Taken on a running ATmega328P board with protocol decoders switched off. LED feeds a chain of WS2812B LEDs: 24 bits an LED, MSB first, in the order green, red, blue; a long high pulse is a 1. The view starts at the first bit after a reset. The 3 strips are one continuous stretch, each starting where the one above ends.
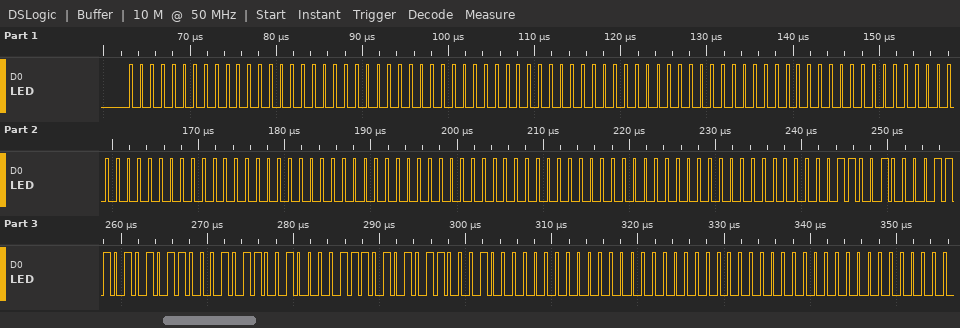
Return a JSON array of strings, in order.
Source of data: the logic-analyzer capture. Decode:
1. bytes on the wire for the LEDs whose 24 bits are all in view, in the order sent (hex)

["00 00 00 00 00 00 00 00 00 00 00 00 00 00 00 00 00 00 64 3A B1 64 3A B1 00 00 00"]
